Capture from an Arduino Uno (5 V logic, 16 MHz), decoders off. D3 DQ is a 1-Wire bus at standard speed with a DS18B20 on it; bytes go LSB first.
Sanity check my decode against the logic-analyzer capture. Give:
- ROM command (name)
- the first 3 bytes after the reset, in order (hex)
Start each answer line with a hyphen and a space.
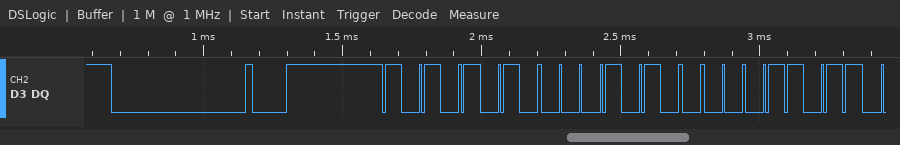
- Match ROM
- 55 28 D8
